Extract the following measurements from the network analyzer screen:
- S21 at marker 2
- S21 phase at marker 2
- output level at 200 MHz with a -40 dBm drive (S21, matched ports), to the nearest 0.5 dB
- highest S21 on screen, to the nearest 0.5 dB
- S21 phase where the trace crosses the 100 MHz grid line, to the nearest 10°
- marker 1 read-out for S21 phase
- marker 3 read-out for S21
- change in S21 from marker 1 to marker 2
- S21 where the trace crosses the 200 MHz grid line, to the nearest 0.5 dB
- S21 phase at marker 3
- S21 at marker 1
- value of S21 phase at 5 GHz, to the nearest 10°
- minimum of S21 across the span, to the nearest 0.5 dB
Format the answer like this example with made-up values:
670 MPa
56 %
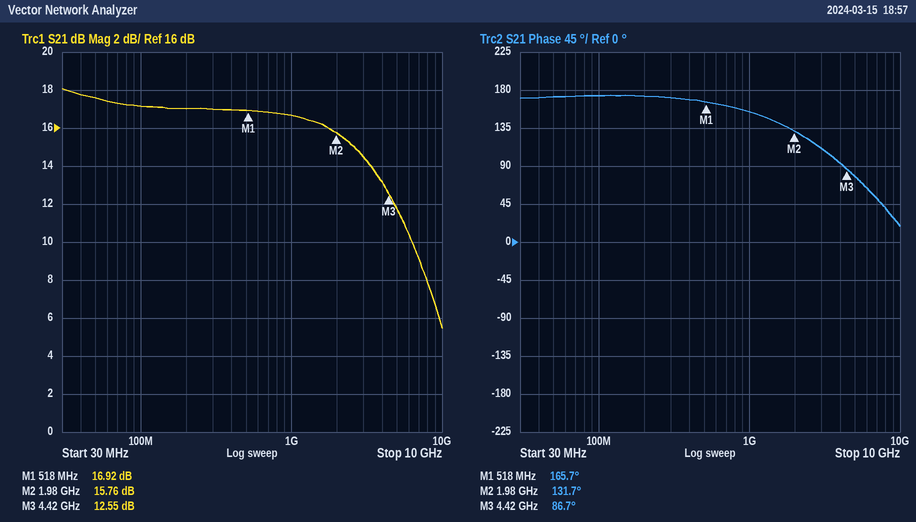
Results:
15.76 dB
131.7°
-23.0 dBm
18.0 dB
170°
165.7°
12.55 dB
-1.16 dB
17.0 dB
86.7°
16.92 dB
80°
5.5 dB
